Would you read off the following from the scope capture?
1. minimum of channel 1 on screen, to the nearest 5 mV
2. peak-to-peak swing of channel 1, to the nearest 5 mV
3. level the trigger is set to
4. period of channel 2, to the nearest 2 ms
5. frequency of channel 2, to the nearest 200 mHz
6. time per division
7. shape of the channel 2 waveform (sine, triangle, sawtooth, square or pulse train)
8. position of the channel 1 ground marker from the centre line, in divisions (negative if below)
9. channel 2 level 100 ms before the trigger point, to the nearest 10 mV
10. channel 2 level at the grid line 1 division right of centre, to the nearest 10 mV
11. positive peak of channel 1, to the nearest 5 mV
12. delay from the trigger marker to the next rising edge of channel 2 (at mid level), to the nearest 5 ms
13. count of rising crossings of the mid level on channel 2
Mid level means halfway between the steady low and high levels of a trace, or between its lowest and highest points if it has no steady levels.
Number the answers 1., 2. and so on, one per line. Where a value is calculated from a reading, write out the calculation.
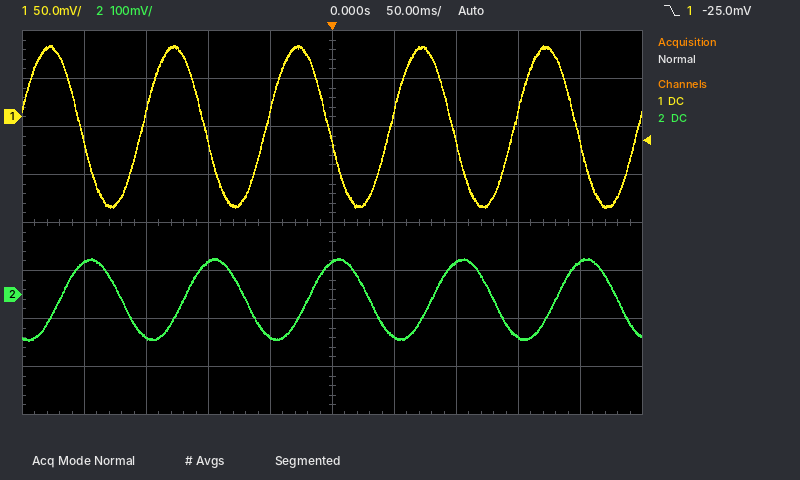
1. -95 mV
2. 75 mV − (-95 mV) = 170 mV
3. -25.0 mV
4. 100 ms
5. 1 / 100 ms ≈ 10.0 Hz
6. 50 ms
7. sine
8. +2.2 div
9. 70 mV
10. -90 mV
11. 75 mV
12. 80 ms
13. 5
